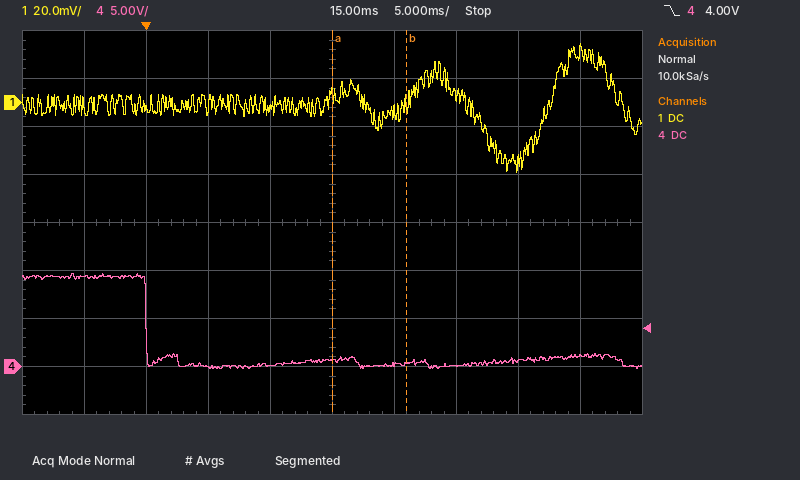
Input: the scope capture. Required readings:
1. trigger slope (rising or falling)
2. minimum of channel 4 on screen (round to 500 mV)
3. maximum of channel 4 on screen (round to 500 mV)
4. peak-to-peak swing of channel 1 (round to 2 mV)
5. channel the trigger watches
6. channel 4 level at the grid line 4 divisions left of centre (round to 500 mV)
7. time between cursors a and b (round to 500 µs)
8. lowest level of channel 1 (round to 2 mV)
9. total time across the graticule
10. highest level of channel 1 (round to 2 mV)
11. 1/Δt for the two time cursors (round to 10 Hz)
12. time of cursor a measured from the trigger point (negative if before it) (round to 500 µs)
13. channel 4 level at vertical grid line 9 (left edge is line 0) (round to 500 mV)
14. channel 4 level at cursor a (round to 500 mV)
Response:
falling
0.0 V
9.5 V
54 mV
channel 4
9.5 V
6.0 ms
-30 mV
50 ms
24 mV
170 Hz
+15.0 ms
1.0 V
500 mV
